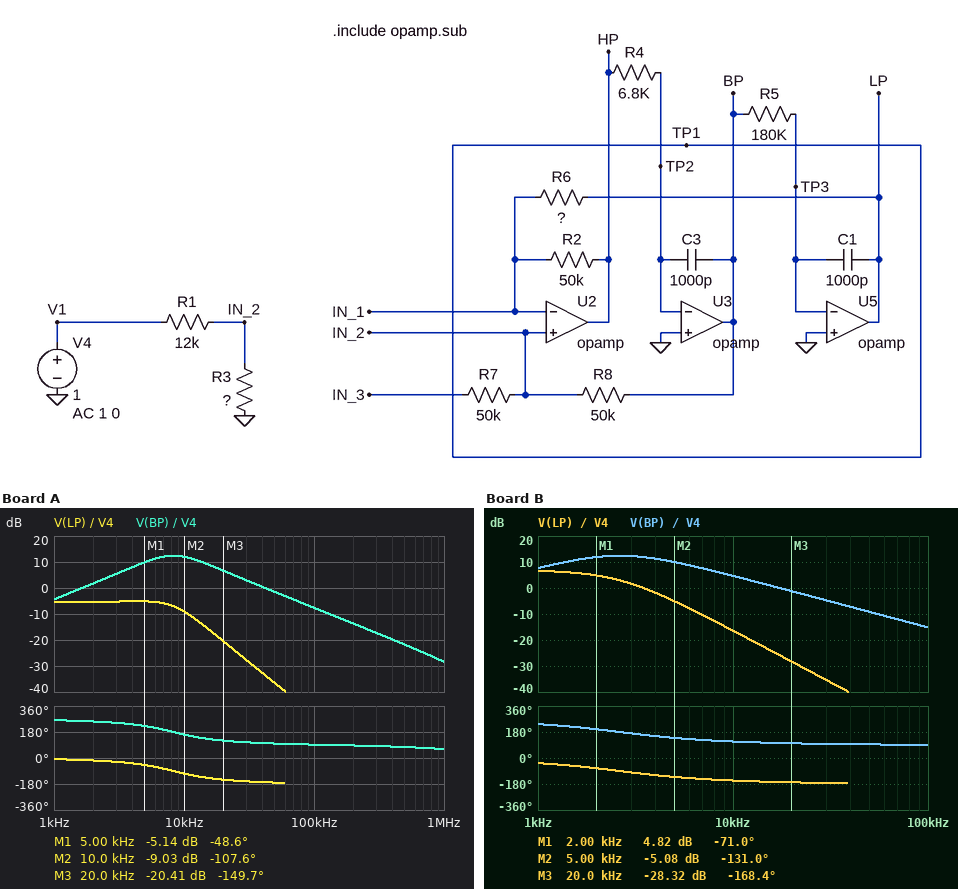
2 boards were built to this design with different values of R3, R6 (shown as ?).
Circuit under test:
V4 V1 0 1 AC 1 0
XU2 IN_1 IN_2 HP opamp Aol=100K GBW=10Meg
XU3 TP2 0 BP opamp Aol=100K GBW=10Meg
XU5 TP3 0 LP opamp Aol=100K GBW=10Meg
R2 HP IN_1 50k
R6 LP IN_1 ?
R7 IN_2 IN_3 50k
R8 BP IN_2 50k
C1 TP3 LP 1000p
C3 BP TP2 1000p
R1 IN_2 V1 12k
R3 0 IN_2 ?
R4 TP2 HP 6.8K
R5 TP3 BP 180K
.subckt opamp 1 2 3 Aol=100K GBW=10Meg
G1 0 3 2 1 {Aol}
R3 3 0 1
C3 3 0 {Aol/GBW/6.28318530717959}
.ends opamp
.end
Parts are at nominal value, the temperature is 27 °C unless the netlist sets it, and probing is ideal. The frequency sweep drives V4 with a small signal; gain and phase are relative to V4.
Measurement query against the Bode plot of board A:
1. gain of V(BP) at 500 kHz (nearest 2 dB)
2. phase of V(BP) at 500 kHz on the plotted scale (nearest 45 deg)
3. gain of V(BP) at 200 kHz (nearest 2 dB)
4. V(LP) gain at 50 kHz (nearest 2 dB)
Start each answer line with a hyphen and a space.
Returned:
- -22 dB
- 90 deg
- -14 dB
- -36 dB
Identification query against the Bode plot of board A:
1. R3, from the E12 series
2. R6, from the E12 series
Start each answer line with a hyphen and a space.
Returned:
- 10 kΩ
- 15 kΩ
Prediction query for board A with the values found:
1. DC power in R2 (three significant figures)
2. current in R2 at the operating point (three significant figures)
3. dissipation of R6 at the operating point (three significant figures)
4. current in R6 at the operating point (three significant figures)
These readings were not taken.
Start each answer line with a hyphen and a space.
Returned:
- 3.36 µW
- 8.20 µA
- 1.01 µW
- 8.20 µA
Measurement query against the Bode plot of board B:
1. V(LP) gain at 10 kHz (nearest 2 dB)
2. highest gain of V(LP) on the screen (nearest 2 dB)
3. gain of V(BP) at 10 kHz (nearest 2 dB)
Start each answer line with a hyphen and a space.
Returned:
- -16 dB
- 6 dB
- 4 dB
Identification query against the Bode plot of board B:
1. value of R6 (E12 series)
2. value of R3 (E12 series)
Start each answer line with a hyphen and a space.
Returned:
- 150 kΩ
- 22 kΩ
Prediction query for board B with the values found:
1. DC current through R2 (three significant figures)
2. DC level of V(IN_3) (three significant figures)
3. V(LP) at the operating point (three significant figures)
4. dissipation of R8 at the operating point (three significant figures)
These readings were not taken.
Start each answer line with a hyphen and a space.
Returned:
- 11.2 µA
- 560 mV
- 2.24 V
- 6.27 µW
